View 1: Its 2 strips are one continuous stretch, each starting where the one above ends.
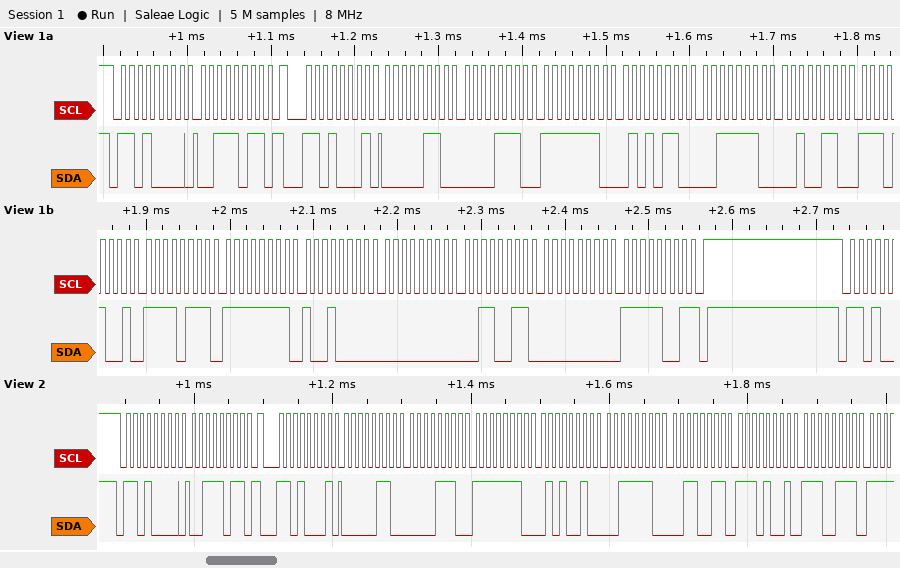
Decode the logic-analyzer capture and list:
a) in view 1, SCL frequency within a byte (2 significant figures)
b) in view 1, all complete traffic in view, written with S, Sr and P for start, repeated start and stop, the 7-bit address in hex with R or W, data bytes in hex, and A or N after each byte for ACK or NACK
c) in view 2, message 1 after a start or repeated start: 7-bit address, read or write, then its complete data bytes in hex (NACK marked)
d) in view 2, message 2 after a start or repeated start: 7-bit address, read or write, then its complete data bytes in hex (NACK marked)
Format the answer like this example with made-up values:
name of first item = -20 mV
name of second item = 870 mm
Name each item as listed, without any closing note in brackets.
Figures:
in view 1, SCL frequency within a byte = 100 kHz
in view 1, all complete traffic in view, written with S, Sr and P for start, repeated start and stop, the 7-bit address in hex with R or W, data bytes in hex, and A or N after each byte for ACK or NACK = S 68W A 3B A Sr 68R A 06 A 0E A FE A 56 A 3E A 26 A E9 A F7 A FF A 90 A 00 A 33 A 00 A F9 N P
in view 2, message 1 after a start or repeated start: 7-bit address, read or write, then its complete data bytes in hex = 0x68 write: 3B
in view 2, message 2 after a start or repeated start: 7-bit address, read or write, then its complete data bytes in hex = 0x68 read: 06 0E FE 52 3E 33 E9 E7
